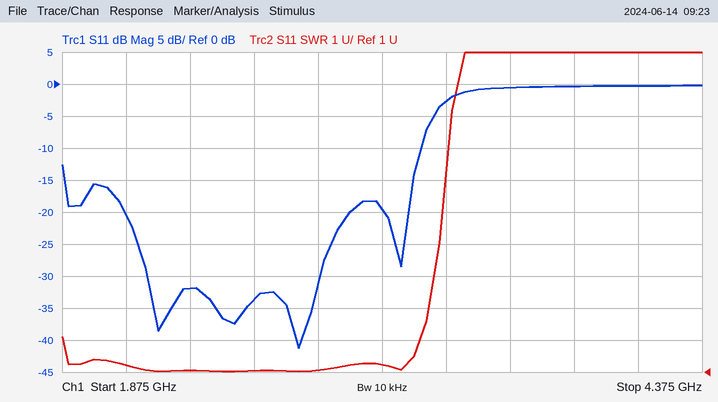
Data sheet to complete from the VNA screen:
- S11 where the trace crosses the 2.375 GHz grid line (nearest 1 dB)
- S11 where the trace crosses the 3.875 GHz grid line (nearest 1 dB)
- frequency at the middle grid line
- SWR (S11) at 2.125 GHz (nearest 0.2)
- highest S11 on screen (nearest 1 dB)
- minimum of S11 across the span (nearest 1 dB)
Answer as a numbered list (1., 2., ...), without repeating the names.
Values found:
1. -32 dB
2. 0 dB
3. 3.125 GHz
4. 1.2
5. 0 dB
6. -41 dB
